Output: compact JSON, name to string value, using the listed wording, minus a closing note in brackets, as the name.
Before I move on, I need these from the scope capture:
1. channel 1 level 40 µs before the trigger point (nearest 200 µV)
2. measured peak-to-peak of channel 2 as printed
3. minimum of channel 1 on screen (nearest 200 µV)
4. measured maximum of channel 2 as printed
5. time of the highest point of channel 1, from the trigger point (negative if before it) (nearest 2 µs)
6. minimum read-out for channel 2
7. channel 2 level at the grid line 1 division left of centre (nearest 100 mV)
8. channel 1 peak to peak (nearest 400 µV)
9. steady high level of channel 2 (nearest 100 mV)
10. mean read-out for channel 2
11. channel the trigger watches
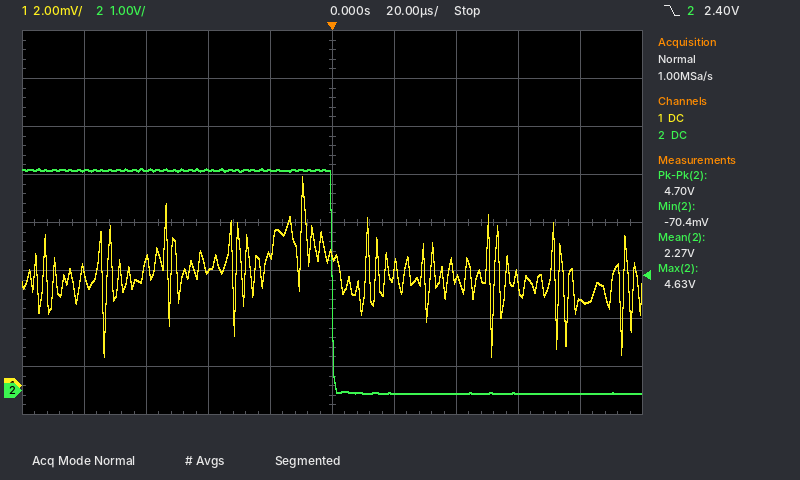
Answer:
{"channel 1 level 40 µs before the trigger point": "4.8 mV", "measured peak-to-peak of channel 2 as printed": "4.70 V", "minimum of channel 1 on screen": "1.2 mV", "measured maximum of channel 2 as printed": "4.63 V", "time of the highest point of channel 1, from the trigger point (negative if before it)": "-10 µs", "minimum read-out for channel 2": "-70.4 mV", "channel 2 level at the grid line 1 division left of centre": "4.6 V", "channel 1 peak to peak": "7.6 mV", "steady high level of channel 2": "4.6 V", "mean read-out for channel 2": "2.27 V", "channel the trigger watches": "channel 2"}
